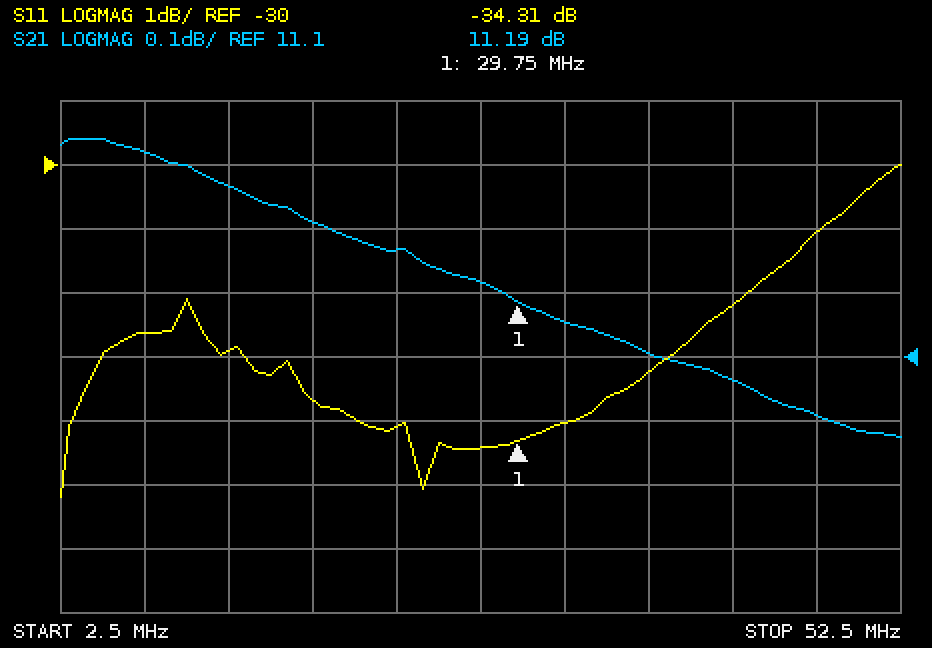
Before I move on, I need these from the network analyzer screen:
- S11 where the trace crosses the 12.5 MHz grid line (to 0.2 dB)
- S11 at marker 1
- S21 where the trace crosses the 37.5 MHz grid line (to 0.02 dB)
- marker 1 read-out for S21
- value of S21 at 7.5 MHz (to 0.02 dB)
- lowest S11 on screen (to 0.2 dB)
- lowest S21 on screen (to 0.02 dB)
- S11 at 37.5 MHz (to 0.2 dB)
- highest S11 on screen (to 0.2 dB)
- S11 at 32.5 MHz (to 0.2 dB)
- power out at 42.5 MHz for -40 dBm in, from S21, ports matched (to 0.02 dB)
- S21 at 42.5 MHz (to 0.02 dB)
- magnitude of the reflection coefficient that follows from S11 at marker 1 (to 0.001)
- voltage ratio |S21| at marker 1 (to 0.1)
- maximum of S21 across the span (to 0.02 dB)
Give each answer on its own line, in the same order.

-33.0 dB
-34.31 dB
11.10 dB
11.19 dB
11.42 dB
-35.2 dB
10.98 dB
-33.2 dB
-30.0 dB
-34.0 dB
-28.94 dBm
11.06 dB
0.019
3.6
11.44 dB
